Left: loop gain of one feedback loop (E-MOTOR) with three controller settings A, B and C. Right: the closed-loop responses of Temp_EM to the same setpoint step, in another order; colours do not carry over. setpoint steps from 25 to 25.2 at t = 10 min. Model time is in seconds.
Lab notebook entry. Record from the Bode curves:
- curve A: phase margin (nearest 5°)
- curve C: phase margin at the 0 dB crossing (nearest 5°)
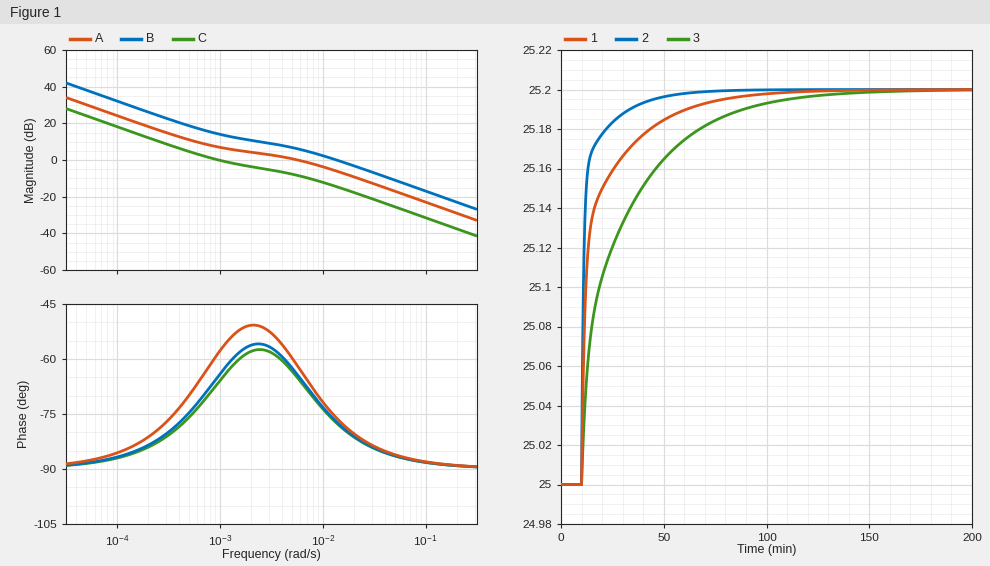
120°
115°
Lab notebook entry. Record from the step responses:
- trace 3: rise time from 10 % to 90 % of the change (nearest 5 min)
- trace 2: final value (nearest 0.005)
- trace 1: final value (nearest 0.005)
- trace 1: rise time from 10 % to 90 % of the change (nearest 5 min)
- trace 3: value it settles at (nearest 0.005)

55 min
25.200
25.200
35 min
25.200
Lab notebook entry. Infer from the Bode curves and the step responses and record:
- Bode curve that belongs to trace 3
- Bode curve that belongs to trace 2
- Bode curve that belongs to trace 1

C
B
A
